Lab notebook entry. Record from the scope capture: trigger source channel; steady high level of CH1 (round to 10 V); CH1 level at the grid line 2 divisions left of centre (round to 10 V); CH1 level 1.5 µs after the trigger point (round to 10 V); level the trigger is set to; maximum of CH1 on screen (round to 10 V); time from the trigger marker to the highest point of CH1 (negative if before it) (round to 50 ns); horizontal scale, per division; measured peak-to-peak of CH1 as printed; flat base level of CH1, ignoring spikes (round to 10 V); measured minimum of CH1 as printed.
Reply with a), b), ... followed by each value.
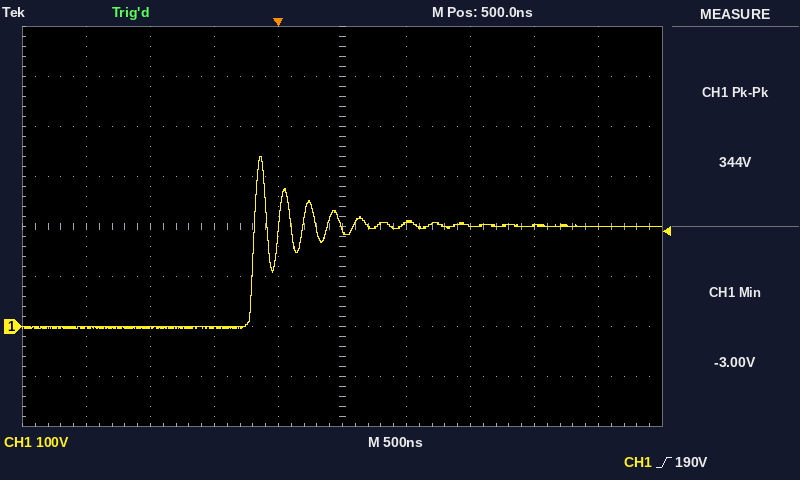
a) CH1
b) 200 V
c) 0 V
d) 200 V
e) 190 V
f) 340 V
g) -150 ns
h) 500 ns
i) 344 V
j) 0 V
k) -3.00 V
